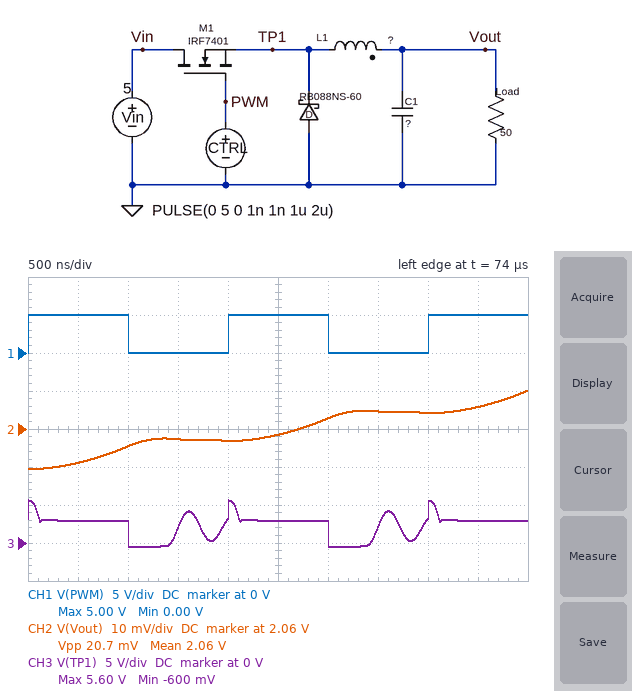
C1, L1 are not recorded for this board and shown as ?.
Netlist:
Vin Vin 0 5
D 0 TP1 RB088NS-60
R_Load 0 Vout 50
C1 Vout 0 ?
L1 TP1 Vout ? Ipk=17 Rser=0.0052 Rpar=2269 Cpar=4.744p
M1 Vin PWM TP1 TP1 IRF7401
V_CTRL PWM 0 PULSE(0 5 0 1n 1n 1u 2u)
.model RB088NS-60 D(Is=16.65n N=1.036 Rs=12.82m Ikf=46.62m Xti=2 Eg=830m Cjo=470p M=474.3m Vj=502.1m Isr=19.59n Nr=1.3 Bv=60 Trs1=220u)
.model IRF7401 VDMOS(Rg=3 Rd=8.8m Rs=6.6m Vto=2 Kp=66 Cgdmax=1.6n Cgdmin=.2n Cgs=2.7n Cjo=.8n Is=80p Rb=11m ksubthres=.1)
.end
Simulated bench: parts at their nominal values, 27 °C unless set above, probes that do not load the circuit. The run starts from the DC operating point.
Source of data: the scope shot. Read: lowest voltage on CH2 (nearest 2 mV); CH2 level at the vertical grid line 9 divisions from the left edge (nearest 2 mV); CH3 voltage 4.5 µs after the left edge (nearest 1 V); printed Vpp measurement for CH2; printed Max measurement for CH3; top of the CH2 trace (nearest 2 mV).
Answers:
2.050 V
2.066 V
3 V
20.7 mV
5.60 V
2.070 V
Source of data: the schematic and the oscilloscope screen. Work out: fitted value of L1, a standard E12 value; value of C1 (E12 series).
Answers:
1.5 µH
56 µF
